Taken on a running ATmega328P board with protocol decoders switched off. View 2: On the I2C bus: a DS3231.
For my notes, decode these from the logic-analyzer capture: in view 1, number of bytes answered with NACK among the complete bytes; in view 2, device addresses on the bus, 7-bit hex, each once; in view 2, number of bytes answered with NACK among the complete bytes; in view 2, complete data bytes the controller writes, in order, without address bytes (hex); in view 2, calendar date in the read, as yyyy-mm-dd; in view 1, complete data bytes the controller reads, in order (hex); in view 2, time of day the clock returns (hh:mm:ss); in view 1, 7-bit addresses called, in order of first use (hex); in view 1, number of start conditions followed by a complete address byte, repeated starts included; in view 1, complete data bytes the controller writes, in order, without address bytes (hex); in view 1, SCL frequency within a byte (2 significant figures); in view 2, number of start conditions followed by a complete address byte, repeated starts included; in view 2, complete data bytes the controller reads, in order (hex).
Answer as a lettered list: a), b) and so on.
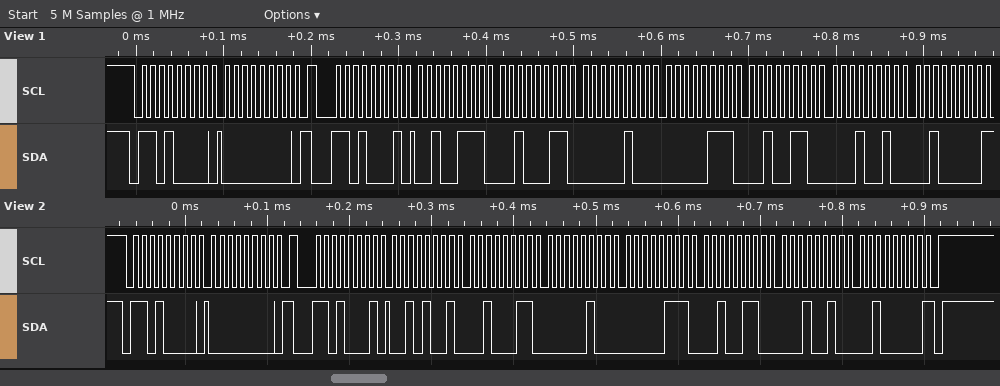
a) 1
b) 0x68
c) 1
d) 00
e) 2020-12-26
f) 27 23 04 07 26 12 20
g) 04:23:29
h) 0x68
i) 2
j) 00
k) 100 kHz
l) 2
m) 29 23 04 07 26 12 20
